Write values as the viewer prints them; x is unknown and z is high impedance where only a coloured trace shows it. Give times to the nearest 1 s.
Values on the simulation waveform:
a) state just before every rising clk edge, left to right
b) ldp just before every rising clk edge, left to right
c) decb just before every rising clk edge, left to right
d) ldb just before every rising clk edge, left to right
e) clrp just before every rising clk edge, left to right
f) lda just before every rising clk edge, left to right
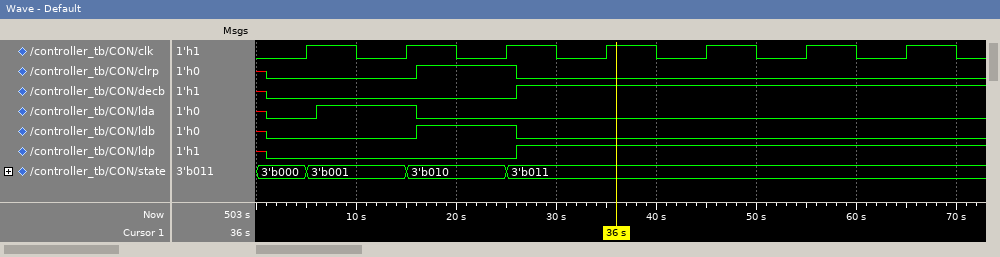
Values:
3'b000, 3'b001, 3'b010, 3'b011, 3'b011, 3'b011, 3'b011
0 0 0 1 1 1 1
0 0 0 1 1 1 1
0 0 1 0 0 0 0
0 0 1 0 0 0 0
0 1 0 0 0 0 0
